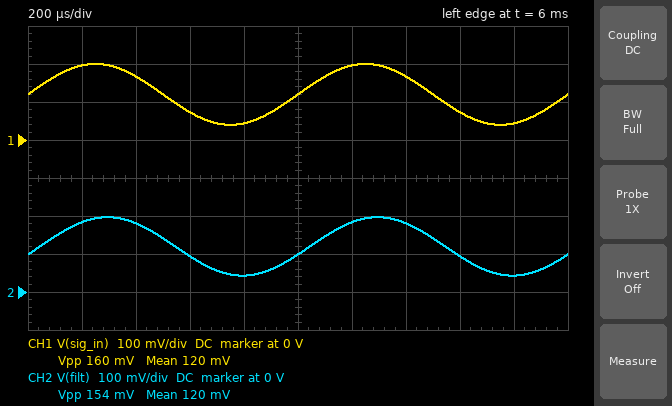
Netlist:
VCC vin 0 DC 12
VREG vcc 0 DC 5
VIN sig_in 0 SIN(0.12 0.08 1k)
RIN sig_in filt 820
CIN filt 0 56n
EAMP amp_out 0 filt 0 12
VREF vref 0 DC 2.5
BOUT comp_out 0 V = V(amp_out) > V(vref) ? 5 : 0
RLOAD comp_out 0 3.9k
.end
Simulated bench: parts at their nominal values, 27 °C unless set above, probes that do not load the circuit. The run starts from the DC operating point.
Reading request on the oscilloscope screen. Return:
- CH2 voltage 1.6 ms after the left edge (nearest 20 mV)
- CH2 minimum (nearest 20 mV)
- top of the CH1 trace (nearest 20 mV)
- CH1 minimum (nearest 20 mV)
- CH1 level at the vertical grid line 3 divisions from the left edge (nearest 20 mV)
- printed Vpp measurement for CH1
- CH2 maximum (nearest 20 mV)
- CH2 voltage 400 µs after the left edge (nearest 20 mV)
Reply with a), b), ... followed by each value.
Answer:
a) 100 mV
b) 40 mV
c) 200 mV
d) 40 mV
e) 80 mV
f) 160 mV
g) 200 mV
h) 180 mV
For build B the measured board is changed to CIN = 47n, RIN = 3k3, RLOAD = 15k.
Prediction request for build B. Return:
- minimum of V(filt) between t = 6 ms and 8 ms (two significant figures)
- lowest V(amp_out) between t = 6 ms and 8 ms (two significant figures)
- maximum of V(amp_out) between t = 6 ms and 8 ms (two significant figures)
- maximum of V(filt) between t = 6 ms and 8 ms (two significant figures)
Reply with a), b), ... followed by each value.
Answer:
a) 63 mV
b) 750 mV
c) 2.1 V
d) 180 mV
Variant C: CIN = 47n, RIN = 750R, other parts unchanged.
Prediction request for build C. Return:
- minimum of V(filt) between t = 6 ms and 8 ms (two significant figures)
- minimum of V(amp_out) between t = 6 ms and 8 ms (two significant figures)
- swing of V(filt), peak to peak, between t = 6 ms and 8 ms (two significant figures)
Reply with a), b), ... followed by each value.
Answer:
a) 42 mV
b) 500 mV
c) 160 mV
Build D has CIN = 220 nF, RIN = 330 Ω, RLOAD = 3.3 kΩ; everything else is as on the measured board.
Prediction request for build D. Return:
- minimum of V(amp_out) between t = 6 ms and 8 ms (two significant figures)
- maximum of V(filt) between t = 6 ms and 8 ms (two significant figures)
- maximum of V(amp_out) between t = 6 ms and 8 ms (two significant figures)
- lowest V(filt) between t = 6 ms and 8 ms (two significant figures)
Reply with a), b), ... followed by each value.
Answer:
a) 570 mV
b) 190 mV
c) 2.3 V
d) 47 mV
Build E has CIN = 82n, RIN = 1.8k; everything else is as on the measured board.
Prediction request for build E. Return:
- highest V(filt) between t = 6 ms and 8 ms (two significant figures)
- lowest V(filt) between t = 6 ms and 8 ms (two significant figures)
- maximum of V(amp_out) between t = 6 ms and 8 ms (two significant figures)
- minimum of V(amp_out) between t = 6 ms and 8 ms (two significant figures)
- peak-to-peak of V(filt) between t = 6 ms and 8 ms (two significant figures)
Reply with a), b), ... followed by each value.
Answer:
a) 180 mV
b) 61 mV
c) 2.1 V
d) 740 mV
e) 120 mV
